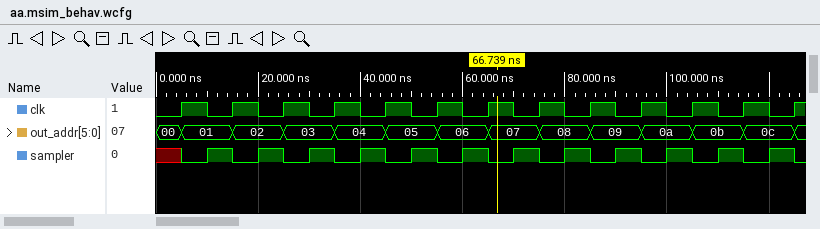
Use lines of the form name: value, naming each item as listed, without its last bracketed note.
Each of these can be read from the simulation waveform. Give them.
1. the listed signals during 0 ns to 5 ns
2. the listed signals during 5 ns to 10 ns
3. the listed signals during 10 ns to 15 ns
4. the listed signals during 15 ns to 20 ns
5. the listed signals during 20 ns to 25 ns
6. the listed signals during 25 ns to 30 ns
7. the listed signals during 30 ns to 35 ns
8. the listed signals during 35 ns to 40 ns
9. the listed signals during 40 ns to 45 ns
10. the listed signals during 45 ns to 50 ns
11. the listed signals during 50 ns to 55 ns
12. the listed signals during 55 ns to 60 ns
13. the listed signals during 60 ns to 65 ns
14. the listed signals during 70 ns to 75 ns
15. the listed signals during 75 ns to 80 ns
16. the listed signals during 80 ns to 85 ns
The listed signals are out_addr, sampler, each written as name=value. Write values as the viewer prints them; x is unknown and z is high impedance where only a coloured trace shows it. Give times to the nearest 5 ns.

the listed signals during 0 ns to 5 ns: out_addr=00, sampler=x
the listed signals during 5 ns to 10 ns: out_addr=01, sampler=0
the listed signals during 10 ns to 15 ns: out_addr=01, sampler=1
the listed signals during 15 ns to 20 ns: out_addr=02, sampler=0
the listed signals during 20 ns to 25 ns: out_addr=02, sampler=1
the listed signals during 25 ns to 30 ns: out_addr=03, sampler=0
the listed signals during 30 ns to 35 ns: out_addr=03, sampler=1
the listed signals during 35 ns to 40 ns: out_addr=04, sampler=0
the listed signals during 40 ns to 45 ns: out_addr=04, sampler=1
the listed signals during 45 ns to 50 ns: out_addr=05, sampler=0
the listed signals during 50 ns to 55 ns: out_addr=05, sampler=1
the listed signals during 55 ns to 60 ns: out_addr=06, sampler=0
the listed signals during 60 ns to 65 ns: out_addr=06, sampler=1
the listed signals during 70 ns to 75 ns: out_addr=07, sampler=1
the listed signals during 75 ns to 80 ns: out_addr=08, sampler=0
the listed signals during 80 ns to 85 ns: out_addr=08, sampler=1
